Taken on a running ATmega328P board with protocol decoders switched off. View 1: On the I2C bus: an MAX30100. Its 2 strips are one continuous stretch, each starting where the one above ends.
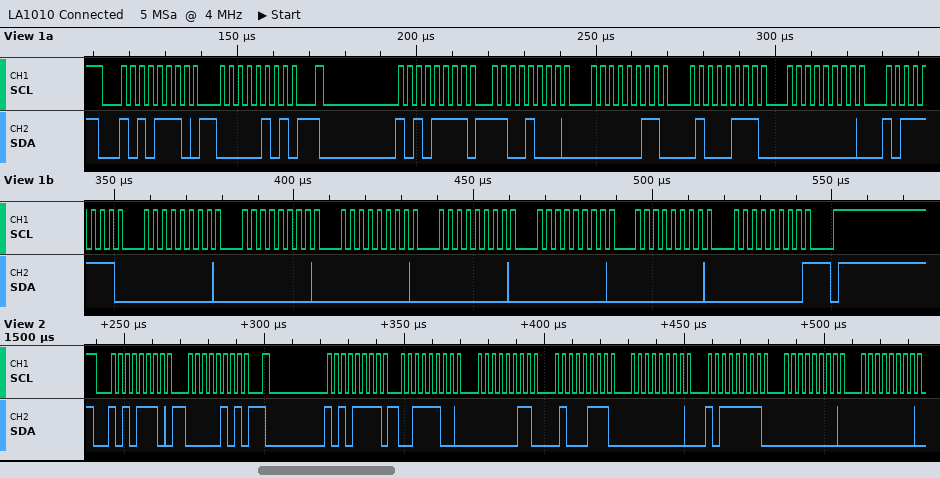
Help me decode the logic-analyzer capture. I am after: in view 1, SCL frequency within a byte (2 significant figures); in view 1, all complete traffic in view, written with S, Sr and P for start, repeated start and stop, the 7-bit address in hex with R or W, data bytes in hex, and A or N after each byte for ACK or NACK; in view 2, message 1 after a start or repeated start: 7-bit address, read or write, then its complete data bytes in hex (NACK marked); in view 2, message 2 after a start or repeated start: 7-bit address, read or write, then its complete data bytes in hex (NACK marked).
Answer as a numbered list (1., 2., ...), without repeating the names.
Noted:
1. 400 kHz
2. S 57W A 05 A Sr 57R A C8 A 03 A 47 A 00 A BF A 00 A 00 A 00 A 00 A 00 A 00 A 00 N P
3. 0x57 write: 05
4. 0x57 read: 3C 03 47 00 BF 00 00
